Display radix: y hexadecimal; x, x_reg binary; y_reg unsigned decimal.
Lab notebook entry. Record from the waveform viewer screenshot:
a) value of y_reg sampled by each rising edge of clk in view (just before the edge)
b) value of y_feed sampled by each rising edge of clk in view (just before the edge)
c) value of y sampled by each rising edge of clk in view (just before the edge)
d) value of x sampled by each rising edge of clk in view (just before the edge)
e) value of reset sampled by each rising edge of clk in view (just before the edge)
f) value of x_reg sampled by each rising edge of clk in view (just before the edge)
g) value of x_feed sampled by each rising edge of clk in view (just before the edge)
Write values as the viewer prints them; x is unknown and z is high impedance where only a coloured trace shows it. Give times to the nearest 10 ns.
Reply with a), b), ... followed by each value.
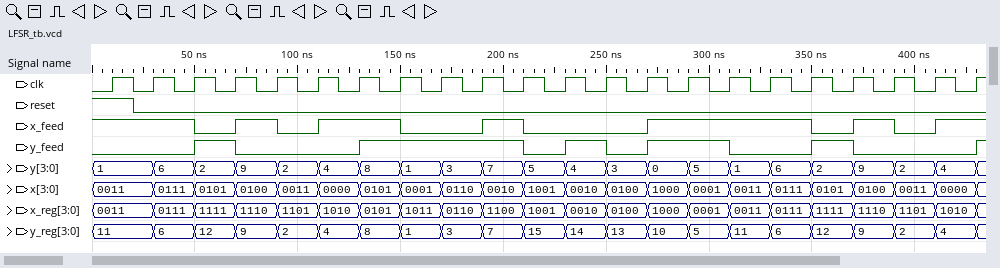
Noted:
a) 11, 11, 6, 12, 9, 2, 4, 8, 1, 3, 7, 15, 14, 13, 10, 5, 11, 6, 12, 9, 2, 4
b) 0 0 0 1 0 0 0 1 1 1 1 0 1 0 1 1 0 0 1 0 0 0
c) 1, 1, 6, 2, 9, 2, 4, 8, 1, 3, 7, 5, 4, 3, 0, 5, 1, 6, 2, 9, 2, 4
d) 0011, 0011, 0111, 0101, 0100, 0011, 0000, 0101, 0001, 0110, 0010, 1001, 0010, 0100, 1000, 0001, 0011, 0111, 0101, 0100, 0011, 0000
e) 1 0 0 0 0 0 0 0 0 0 0 0 0 0 0 0 0 0 0 0 0 0
f) 0011, 0011, 0111, 1111, 1110, 1101, 1010, 0101, 1011, 0110, 1100, 1001, 0010, 0100, 1000, 0001, 0011, 0111, 1111, 1110, 1101, 1010
g) 1 1 1 0 1 0 1 1 0 0 1 0 0 0 1 1 1 1 0 1 0 1
